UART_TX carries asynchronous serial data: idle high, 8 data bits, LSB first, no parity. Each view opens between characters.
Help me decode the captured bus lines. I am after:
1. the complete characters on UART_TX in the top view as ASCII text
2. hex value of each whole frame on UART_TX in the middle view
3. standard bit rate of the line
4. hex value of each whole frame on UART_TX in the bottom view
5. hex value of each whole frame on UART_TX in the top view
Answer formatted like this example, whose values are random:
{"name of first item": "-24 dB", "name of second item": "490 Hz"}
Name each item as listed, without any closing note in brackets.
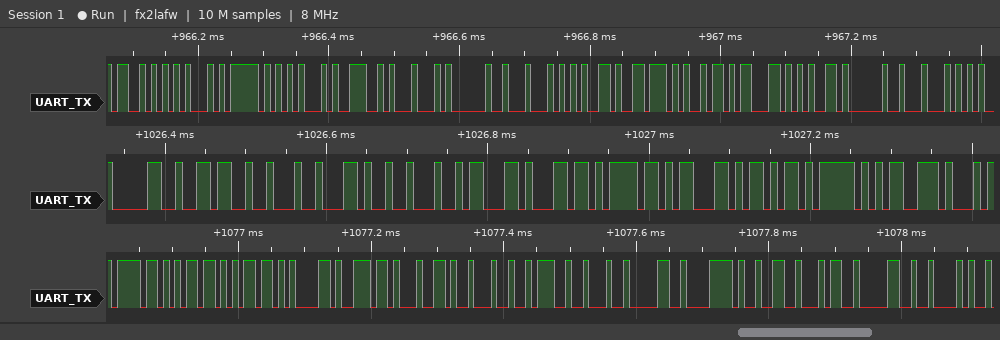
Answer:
{"the complete characters on UART_TX in the top view as ASCII text": "\"SE_END Device D\"", "hex value of each whole frame on UART_TX in the middle view": "30, 36, 22, 2C, 22, 63, 6C, 6F, 63, 6B, 5F, 73", "standard bit rate of the line": "115200 baud", "hex value of each whole frame on UART_TX in the bottom view": "6F, 6D, 6D, 61, 6E, 64, 22, 3A, 22, 30, 78, 32, 34, 30, 42", "hex value of each whole frame on UART_TX in the top view": "53, 45, 5F, 45, 4E, 44, 20, 44, 65, 76, 69, 63, 65, 20, 44"}
